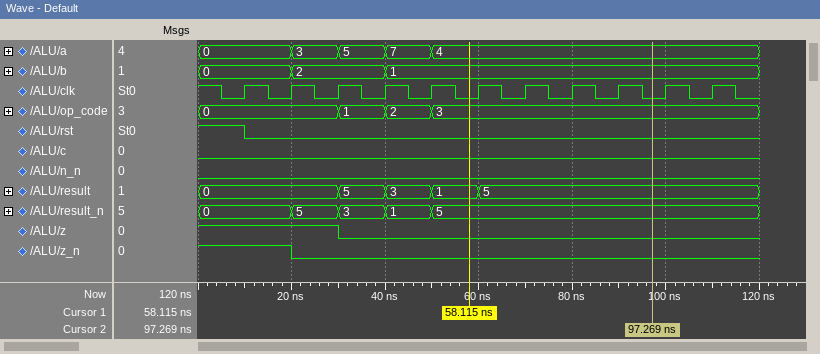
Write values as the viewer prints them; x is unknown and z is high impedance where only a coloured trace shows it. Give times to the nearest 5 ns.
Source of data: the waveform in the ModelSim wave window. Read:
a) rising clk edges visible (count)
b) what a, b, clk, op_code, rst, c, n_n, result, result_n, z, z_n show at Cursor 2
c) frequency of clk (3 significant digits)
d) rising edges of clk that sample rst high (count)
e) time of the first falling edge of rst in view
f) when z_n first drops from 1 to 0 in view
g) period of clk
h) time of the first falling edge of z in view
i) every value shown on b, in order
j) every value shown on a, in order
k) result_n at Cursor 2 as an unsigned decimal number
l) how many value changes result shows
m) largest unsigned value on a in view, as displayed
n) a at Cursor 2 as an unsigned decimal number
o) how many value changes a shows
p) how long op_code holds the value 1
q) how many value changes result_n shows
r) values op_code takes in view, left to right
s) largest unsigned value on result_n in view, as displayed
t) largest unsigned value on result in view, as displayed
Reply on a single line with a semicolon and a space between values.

11; a=4, b=1, clk=0, op_code=3, rst=0, c=0, n_n=0, result=5, result_n=5, z=0, z_n=0; 100 MHz; 1; 10 ns; 20 ns; 10 ns; 30 ns; 0, 2, 1; 0, 3, 5, 7, 4; 5; 4; 7; 4; 4; 10 ns; 4; 0, 1, 2, 3; 5; 5
